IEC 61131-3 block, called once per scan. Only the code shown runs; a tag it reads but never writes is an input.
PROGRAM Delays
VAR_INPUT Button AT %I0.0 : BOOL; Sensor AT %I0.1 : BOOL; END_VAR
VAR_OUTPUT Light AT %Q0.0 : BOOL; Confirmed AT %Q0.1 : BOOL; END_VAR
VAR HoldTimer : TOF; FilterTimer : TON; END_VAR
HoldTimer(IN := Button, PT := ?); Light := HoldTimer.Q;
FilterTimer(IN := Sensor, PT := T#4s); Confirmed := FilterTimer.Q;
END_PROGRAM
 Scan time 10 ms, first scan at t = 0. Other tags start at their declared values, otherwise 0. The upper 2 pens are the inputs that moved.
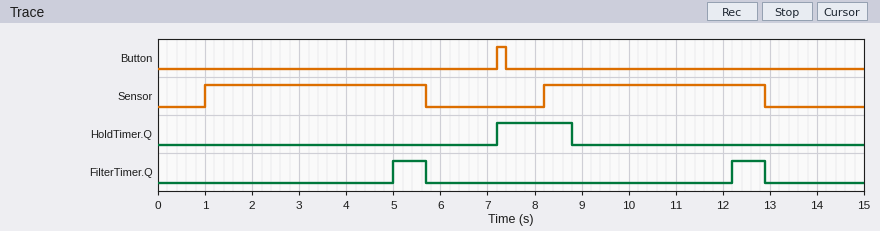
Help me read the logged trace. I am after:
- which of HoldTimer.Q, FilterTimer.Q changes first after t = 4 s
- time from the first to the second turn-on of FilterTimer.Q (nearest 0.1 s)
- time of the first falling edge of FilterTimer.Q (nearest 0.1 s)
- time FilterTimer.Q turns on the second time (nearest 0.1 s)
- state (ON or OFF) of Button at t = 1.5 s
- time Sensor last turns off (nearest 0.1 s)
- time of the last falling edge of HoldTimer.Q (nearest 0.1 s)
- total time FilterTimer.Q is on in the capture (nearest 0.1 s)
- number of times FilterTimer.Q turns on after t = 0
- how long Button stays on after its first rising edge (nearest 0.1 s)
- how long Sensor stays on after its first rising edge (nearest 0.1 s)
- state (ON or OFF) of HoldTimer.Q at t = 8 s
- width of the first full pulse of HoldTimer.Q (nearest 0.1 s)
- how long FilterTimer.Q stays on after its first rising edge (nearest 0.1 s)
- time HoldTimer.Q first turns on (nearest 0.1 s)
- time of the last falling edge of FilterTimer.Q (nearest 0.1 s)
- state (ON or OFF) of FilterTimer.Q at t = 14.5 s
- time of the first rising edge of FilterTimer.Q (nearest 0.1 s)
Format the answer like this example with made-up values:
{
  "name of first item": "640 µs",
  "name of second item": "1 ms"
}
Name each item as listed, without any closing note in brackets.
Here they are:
{
  "which of HoldTimer.Q, FilterTimer.Q changes first after t = 4 s": "FilterTimer.Q",
  "time from the first to the second turn-on of FilterTimer.Q": "7.2 s",
  "time of the first falling edge of FilterTimer.Q": "5.7 s",
  "time FilterTimer.Q turns on the second time": "12.2 s",
  "state (ON or OFF) of Button at t = 1.5 s": "OFF",
  "time Sensor last turns off": "12.9 s",
  "time of the last falling edge of HoldTimer.Q": "8.8 s",
  "total time FilterTimer.Q is on in the capture": "1.4 s",
  "number of times FilterTimer.Q turns on after t = 0": "2",
  "how long Button stays on after its first rising edge": "0.2 s",
  "how long Sensor stays on after its first rising edge": "4.7 s",
  "state (ON or OFF) of HoldTimer.Q at t = 8 s": "ON",
  "width of the first full pulse of HoldTimer.Q": "1.6 s",
  "how long FilterTimer.Q stays on after its first rising edge": "0.7 s",
  "time HoldTimer.Q first turns on": "7.2 s",
  "time of the last falling edge of FilterTimer.Q": "12.9 s",
  "state (ON or OFF) of FilterTimer.Q at t = 14.5 s": "OFF",
  "time of the first rising edge of FilterTimer.Q": "5.0 s"
}
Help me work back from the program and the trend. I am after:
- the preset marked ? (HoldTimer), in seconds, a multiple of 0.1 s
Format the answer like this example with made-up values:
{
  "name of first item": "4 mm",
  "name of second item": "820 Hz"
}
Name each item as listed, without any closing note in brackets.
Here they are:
{
  "the preset marked ? (HoldTimer), in seconds, a multiple of 0.1 s": "1.4 s"
}
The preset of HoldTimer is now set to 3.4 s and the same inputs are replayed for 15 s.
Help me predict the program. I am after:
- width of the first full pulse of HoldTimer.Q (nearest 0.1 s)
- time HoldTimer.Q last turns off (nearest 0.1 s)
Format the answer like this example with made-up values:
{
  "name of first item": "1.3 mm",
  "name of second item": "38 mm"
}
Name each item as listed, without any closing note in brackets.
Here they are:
{
  "width of the first full pulse of HoldTimer.Q": "3.6 s",
  "time HoldTimer.Q last turns off": "10.8 s"
}
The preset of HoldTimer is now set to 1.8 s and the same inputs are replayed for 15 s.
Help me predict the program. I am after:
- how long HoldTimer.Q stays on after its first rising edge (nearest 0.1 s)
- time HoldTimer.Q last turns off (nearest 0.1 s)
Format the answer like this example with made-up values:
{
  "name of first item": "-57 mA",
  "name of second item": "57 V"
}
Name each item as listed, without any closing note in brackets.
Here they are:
{
  "how long HoldTimer.Q stays on after its first rising edge": "2.0 s",
  "time HoldTimer.Q last turns off": "9.2 s"
}
